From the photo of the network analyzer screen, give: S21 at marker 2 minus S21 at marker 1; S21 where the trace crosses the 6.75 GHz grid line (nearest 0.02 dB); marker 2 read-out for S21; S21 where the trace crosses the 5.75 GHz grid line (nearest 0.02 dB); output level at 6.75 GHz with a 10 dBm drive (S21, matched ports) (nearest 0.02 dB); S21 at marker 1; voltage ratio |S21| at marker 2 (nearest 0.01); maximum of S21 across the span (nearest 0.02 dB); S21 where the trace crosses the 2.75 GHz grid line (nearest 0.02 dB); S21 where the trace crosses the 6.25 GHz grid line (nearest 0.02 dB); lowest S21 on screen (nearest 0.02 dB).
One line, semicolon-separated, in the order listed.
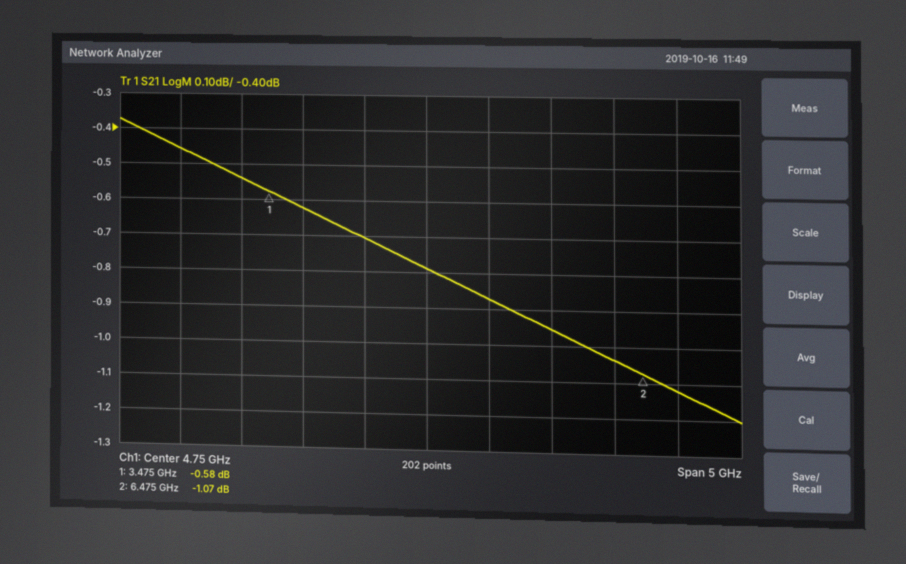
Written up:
-0.49 dB; -1.12 dB; -1.07 dB; -0.96 dB; 8.88 dBm; -0.58 dB; 0.88; -0.38 dB; -0.46 dB; -1.04 dB; -1.20 dB
